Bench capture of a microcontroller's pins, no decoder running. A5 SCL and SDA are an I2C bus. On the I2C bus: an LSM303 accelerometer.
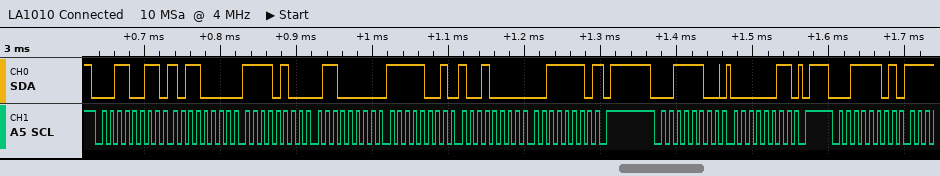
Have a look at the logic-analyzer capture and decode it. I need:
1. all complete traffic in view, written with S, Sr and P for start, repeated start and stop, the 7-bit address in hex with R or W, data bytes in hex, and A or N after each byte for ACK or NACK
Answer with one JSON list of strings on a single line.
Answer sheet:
["S 19R A B0 A F4 A 60 A F9 A 90 A 3E N P S 1EW A 03 A P S 1ER A"]
